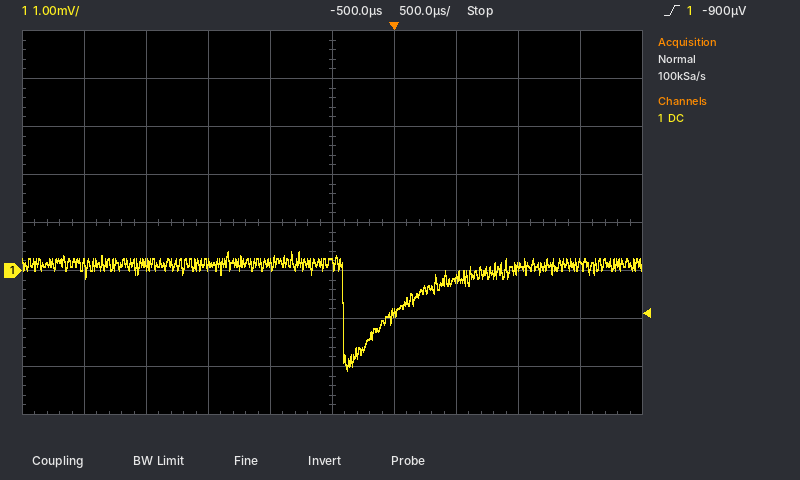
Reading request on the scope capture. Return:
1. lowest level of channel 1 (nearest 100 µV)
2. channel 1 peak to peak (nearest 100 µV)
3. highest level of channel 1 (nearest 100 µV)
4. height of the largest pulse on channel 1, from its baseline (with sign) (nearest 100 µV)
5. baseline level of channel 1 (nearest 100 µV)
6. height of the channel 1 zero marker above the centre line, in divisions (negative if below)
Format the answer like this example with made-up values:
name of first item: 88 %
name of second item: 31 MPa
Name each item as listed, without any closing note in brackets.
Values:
lowest level of channel 1: -2.1 mV
channel 1 peak to peak: 2.5 mV
highest level of channel 1: 400 µV
height of the largest pulse on channel 1, from its baseline (with sign): -2.2 mV
baseline level of channel 1: 100 µV
height of the channel 1 zero marker above the centre line, in divisions: -1.0 div
